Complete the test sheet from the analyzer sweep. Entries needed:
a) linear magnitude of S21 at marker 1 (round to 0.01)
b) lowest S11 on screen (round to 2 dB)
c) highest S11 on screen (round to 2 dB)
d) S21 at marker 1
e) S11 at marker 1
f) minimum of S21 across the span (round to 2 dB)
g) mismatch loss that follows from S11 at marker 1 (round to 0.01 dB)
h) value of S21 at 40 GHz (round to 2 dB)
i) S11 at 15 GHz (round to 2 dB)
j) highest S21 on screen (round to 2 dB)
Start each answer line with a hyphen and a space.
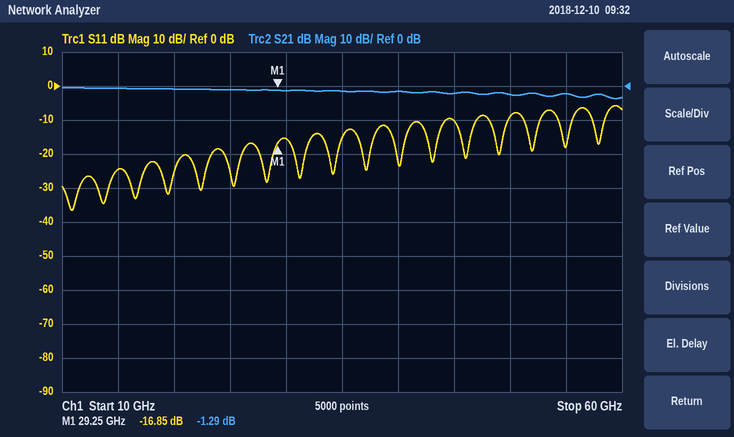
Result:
- 0.86
- -36 dB
- -6 dB
- -1.29 dB
- -16.85 dB
- -4 dB
- 0.09 dB
- -2 dB
- -24 dB
- 0 dB
